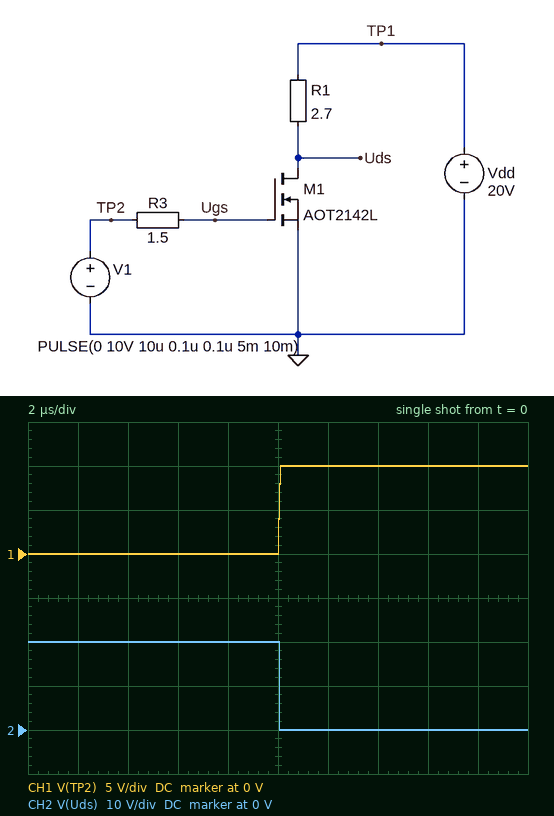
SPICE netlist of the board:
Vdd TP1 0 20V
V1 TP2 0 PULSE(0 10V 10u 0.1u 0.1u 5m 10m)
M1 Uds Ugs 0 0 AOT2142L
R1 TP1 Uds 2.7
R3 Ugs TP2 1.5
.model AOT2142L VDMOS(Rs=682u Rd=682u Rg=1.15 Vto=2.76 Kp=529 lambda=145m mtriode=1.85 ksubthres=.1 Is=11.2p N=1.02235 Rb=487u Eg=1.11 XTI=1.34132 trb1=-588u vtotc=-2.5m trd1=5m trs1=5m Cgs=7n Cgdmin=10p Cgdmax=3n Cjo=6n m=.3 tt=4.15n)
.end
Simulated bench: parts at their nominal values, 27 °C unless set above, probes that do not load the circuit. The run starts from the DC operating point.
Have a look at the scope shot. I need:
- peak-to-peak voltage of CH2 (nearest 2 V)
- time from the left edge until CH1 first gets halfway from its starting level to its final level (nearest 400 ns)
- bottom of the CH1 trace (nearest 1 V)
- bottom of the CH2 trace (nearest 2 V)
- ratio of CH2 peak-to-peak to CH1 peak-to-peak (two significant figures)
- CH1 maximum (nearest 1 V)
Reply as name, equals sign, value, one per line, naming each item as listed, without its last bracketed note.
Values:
peak-to-peak voltage of CH2 = 20 V
time from the left edge until CH1 first gets halfway from its starting level to its final level = 10.0 µs
bottom of the CH1 trace = 0 V
bottom of the CH2 trace = 0 V
ratio of CH2 peak-to-peak to CH1 peak-to-peak = 2.0
CH1 maximum = 10 V
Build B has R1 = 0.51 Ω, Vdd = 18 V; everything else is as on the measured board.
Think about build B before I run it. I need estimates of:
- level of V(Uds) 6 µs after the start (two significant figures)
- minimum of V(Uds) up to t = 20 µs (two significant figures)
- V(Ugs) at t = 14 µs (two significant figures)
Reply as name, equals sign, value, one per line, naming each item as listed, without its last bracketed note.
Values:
level of V(Uds) 6 µs after the start = 18 V
minimum of V(Uds) up to t = 20 µs = 53 mV
V(Ugs) at t = 14 µs = 10 V
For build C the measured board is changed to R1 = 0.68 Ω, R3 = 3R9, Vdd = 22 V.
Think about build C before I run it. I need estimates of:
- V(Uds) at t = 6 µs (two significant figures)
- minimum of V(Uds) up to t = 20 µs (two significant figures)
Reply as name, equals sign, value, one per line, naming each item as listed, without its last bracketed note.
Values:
V(Uds) at t = 6 µs = 22 V
minimum of V(Uds) up to t = 20 µs = 49 mV
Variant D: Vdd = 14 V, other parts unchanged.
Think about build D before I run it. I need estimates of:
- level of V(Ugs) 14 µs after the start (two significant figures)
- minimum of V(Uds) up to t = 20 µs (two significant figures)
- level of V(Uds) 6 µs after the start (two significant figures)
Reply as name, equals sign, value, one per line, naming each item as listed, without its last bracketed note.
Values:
level of V(Ugs) 14 µs after the start = 10 V
minimum of V(Uds) up to t = 20 µs = 7.8 mV
level of V(Uds) 6 µs after the start = 14 V
